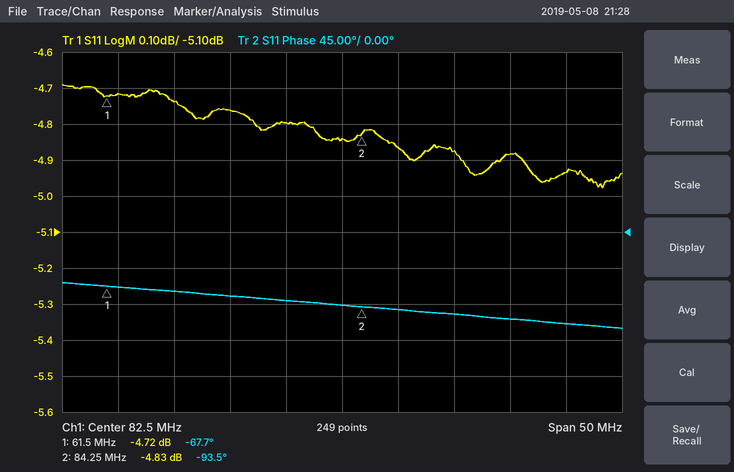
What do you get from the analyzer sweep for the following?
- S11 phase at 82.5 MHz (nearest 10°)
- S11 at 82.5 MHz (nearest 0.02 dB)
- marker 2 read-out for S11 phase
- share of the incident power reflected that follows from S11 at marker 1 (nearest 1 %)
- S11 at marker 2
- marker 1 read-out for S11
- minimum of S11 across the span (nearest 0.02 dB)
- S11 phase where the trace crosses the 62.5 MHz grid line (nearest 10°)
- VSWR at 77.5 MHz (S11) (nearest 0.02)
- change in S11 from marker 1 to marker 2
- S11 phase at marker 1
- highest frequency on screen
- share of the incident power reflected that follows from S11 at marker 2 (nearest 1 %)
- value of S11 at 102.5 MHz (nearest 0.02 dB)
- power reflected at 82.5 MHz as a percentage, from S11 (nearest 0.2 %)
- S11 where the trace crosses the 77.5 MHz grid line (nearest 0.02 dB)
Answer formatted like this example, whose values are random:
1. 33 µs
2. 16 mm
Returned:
1. -90°
2. -4.84 dB
3. -93.5°
4. 34 %
5. -4.83 dB
6. -4.72 dB
7. -4.98 dB
8. -70°
9. 3.72
10. -0.11 dB
11. -67.7°
12. 107.5 MHz
13. 33 %
14. -4.94 dB
15. 32.8 %
16. -4.80 dB
